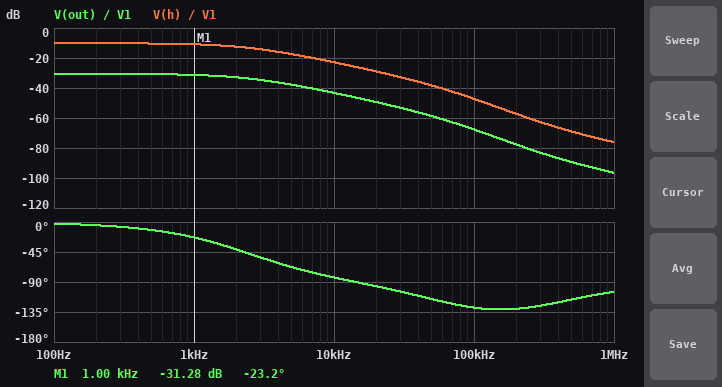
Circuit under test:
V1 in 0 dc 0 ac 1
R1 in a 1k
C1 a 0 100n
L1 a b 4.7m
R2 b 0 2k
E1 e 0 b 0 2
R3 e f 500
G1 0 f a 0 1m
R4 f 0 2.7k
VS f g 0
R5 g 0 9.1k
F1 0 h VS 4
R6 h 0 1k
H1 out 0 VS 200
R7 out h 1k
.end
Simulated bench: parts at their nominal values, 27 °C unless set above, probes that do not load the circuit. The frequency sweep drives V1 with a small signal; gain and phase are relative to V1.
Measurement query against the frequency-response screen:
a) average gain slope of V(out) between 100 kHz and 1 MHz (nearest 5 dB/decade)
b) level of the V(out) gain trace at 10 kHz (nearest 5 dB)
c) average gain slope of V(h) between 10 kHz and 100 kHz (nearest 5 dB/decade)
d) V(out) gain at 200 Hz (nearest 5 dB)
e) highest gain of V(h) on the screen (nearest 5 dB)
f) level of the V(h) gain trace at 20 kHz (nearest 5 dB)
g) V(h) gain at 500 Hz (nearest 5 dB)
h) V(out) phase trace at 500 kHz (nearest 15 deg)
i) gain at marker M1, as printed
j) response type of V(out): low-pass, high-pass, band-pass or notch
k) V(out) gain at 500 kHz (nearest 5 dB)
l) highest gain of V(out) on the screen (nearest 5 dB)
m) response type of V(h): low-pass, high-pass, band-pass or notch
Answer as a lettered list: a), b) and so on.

a) -30 dB/decade
b) -45 dB
c) -25 dB/decade
d) -30 dB
e) -10 dB
f) -30 dB
g) -10 dB
h) -120 deg
i) -31.28 dB
j) low-pass
k) -90 dB
l) -30 dB
m) low-pass
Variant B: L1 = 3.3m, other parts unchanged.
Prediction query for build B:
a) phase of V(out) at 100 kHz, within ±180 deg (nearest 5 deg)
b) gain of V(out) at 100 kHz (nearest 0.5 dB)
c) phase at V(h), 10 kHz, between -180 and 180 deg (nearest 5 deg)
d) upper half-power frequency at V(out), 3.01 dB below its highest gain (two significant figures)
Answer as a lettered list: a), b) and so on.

a) -125 deg
b) -66.0 dB
c) -80 deg
d) 2.4 kHz
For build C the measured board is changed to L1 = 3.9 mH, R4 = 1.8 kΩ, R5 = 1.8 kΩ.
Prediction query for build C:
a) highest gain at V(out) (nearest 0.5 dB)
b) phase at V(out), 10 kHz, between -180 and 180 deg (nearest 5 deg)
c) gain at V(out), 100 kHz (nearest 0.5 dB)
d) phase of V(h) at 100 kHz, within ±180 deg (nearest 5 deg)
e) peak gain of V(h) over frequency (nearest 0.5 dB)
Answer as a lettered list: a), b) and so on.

a) -18.5 dB
b) -80 deg
c) -54.5 dB
d) -125 deg
e) 2.0 dB
